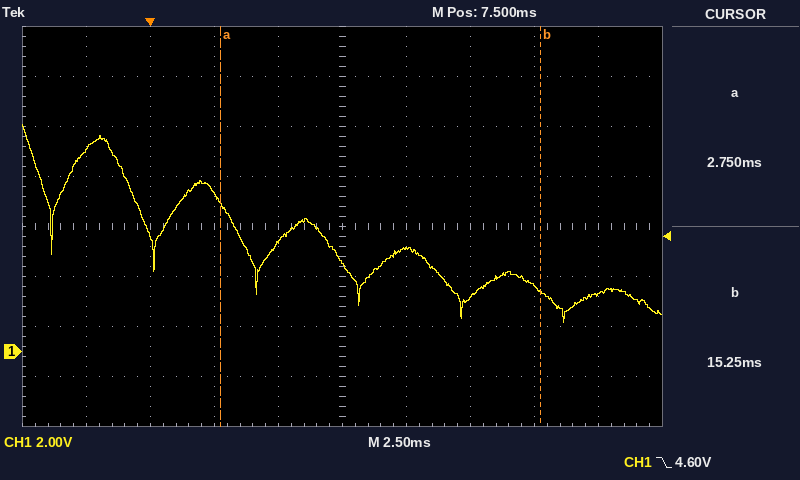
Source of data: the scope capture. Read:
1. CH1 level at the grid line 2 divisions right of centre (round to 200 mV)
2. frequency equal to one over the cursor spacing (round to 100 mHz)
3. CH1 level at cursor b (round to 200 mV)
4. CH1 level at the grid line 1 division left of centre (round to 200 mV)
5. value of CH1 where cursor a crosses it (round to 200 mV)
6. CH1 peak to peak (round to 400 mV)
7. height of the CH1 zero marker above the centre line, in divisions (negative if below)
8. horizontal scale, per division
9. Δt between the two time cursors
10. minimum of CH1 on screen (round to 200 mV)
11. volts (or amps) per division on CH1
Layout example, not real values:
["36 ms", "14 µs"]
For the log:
["2.2 V", "80.0 Hz", "2.4 V", "4.4 V", "6.0 V", "8.0 V", "-2.5 div", "2.5 ms", "12.50 ms", "1.2 V", "2 V"]
